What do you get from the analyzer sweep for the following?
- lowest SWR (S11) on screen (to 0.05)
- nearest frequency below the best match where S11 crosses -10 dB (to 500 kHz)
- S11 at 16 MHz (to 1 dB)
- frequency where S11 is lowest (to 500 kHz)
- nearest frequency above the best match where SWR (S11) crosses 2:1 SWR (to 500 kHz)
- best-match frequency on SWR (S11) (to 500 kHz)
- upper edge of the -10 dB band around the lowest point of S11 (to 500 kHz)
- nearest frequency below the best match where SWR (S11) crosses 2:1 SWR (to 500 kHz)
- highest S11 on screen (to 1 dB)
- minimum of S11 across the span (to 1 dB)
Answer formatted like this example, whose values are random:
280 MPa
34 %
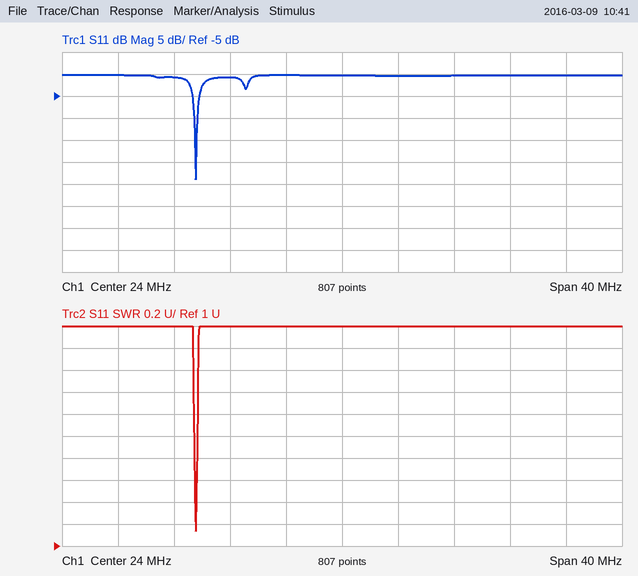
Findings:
1.15
13.5 MHz
-1 dB
13.5 MHz
13.5 MHz
13.5 MHz
13.5 MHz
13.5 MHz
0 dB
-24 dB
